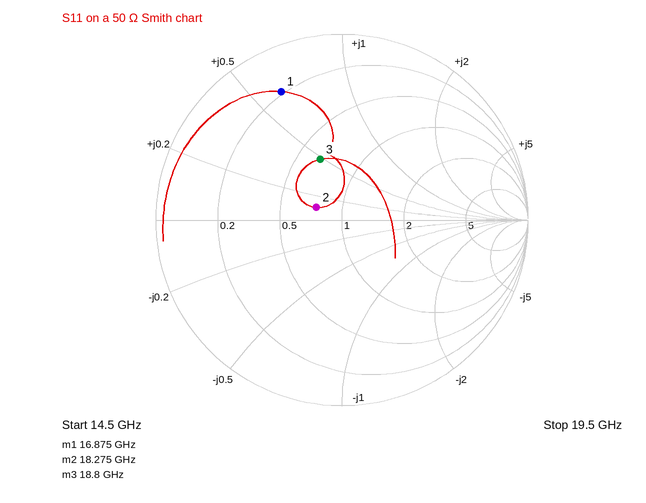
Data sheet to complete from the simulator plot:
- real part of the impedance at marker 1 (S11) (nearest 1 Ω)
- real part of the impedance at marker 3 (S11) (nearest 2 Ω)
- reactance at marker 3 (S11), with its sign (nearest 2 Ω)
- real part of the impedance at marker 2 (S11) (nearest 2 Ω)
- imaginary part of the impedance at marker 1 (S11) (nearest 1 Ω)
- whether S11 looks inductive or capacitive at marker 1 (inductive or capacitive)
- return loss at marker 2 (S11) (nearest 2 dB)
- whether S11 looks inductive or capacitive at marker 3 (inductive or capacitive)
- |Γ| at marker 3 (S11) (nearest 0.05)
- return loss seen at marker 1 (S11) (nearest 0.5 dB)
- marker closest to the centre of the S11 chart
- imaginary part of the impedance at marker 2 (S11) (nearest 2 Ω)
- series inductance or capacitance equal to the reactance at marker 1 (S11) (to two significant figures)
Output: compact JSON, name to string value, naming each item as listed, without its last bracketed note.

{"real part of the impedance at marker 1 (S11)": "9 Ω", "real part of the impedance at marker 3 (S11)": "32 Ω", "reactance at marker 3 (S11), with its sign": "+24 Ω", "real part of the impedance at marker 2 (S11)": "38 Ω", "imaginary part of the impedance at marker 1 (S11)": "+31 Ω", "whether S11 looks inductive or capacitive at marker 1": "inductive", "return loss at marker 2 (S11)": "16 dB", "whether S11 looks inductive or capacitive at marker 3": "inductive", "|Γ| at marker 3 (S11)": "0.35", "return loss seen at marker 1 (S11)": "2.5 dB", "marker closest to the centre of the S11 chart": "marker 2", "imaginary part of the impedance at marker 2 (S11)": "+6 Ω", "series inductance or capacitance equal to the reactance at marker 1 (S11)": "290 pH"}
